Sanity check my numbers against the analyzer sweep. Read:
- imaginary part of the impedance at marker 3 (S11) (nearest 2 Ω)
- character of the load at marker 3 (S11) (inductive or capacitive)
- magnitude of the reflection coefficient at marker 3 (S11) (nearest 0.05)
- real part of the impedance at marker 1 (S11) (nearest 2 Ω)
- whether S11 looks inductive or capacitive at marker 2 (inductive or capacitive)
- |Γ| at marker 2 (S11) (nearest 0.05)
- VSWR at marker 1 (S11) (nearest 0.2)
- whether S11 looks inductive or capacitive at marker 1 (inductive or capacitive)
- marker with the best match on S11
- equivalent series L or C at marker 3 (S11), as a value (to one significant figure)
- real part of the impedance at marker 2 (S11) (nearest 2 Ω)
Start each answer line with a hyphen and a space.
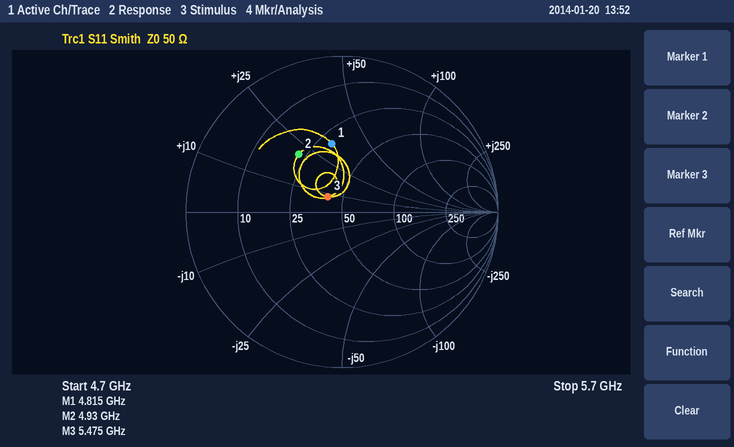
- +8 Ω
- inductive
- 0.15
- 30 Ω
- inductive
- 0.45
- 2.6
- inductive
- marker 3
- 200 pH
- 22 Ω
